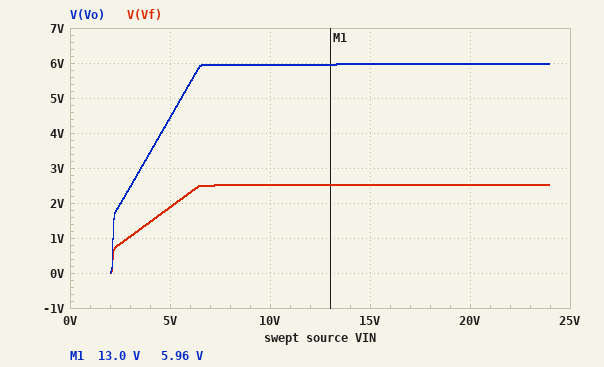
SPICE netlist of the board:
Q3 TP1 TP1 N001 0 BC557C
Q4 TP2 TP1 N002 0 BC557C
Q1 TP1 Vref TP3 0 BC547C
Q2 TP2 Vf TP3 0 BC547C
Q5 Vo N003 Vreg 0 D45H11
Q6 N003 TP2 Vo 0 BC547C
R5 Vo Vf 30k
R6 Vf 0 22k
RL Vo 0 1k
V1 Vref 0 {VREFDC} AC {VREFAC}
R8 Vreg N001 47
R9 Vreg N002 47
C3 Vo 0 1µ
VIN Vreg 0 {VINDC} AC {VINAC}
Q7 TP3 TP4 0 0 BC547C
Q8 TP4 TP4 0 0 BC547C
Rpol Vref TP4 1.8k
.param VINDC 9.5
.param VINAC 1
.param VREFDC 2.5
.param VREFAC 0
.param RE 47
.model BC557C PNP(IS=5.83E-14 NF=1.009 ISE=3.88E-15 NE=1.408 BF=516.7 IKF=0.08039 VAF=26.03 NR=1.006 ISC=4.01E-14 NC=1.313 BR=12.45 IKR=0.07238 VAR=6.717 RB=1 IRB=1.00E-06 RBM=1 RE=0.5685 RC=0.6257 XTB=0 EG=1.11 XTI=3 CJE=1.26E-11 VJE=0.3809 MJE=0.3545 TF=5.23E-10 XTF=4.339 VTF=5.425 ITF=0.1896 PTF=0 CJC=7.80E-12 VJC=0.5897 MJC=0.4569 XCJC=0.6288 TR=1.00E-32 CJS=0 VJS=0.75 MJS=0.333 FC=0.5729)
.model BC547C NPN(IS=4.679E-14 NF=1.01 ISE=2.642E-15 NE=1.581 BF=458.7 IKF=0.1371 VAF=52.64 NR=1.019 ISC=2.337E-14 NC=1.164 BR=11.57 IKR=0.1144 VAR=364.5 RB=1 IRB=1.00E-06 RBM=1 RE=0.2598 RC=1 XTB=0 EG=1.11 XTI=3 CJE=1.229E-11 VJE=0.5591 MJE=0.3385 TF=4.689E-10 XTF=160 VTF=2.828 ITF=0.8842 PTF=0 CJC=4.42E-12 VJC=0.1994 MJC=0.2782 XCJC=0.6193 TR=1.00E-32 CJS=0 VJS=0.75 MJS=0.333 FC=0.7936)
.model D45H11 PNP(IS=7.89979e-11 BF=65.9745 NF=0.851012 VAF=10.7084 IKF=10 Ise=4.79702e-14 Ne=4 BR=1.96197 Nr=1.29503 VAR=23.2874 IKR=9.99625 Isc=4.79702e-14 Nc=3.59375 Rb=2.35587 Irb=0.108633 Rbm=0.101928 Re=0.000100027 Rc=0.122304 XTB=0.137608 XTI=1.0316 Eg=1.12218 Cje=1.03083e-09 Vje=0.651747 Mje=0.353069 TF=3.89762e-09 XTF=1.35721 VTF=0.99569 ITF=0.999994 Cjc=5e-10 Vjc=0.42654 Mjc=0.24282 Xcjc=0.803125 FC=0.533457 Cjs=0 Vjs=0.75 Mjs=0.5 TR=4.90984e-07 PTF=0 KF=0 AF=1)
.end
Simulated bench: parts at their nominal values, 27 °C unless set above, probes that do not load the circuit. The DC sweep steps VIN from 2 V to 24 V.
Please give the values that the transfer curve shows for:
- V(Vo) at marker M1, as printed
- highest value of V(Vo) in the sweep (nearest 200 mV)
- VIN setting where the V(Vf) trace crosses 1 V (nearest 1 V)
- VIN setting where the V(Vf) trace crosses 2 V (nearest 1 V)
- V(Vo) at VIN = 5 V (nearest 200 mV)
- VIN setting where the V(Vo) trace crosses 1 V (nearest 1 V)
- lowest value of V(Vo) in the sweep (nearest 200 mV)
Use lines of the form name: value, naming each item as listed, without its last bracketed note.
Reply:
V(Vo) at marker M1, as printed: 5.96 V
highest value of V(Vo) in the sweep: 6.0 V
VIN setting where the V(Vf) trace crosses 1 V: 3 V
VIN setting where the V(Vf) trace crosses 2 V: 5 V
V(Vo) at VIN = 5 V: 4.4 V
VIN setting where the V(Vo) trace crosses 1 V: 2 V
lowest value of V(Vo) in the sweep: 0 V
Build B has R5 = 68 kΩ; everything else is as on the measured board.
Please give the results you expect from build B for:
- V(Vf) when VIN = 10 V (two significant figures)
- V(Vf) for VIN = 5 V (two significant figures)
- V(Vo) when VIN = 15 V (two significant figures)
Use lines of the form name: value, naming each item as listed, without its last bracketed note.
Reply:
V(Vf) when VIN = 10 V: 2.3 V
V(Vf) for VIN = 5 V: 1.1 V
V(Vo) when VIN = 15 V: 10 V
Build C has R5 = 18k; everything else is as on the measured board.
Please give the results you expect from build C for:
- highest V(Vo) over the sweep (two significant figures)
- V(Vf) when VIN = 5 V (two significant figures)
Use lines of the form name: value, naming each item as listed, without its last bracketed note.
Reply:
highest V(Vo) over the sweep: 4.6 V
V(Vf) when VIN = 5 V: 2.4 V
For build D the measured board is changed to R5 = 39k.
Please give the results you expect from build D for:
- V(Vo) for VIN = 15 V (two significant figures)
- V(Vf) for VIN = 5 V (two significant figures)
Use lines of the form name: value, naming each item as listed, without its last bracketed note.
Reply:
V(Vo) for VIN = 15 V: 7.0 V
V(Vf) for VIN = 5 V: 1.6 V
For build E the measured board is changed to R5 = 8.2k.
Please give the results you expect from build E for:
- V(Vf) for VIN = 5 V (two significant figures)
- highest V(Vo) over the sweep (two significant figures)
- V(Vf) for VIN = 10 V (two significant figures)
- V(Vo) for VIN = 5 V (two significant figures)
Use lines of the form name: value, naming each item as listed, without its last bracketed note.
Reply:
V(Vf) for VIN = 5 V: 2.5 V
highest V(Vo) over the sweep: 3.5 V
V(Vf) for VIN = 10 V: 2.5 V
V(Vo) for VIN = 5 V: 3.4 V
